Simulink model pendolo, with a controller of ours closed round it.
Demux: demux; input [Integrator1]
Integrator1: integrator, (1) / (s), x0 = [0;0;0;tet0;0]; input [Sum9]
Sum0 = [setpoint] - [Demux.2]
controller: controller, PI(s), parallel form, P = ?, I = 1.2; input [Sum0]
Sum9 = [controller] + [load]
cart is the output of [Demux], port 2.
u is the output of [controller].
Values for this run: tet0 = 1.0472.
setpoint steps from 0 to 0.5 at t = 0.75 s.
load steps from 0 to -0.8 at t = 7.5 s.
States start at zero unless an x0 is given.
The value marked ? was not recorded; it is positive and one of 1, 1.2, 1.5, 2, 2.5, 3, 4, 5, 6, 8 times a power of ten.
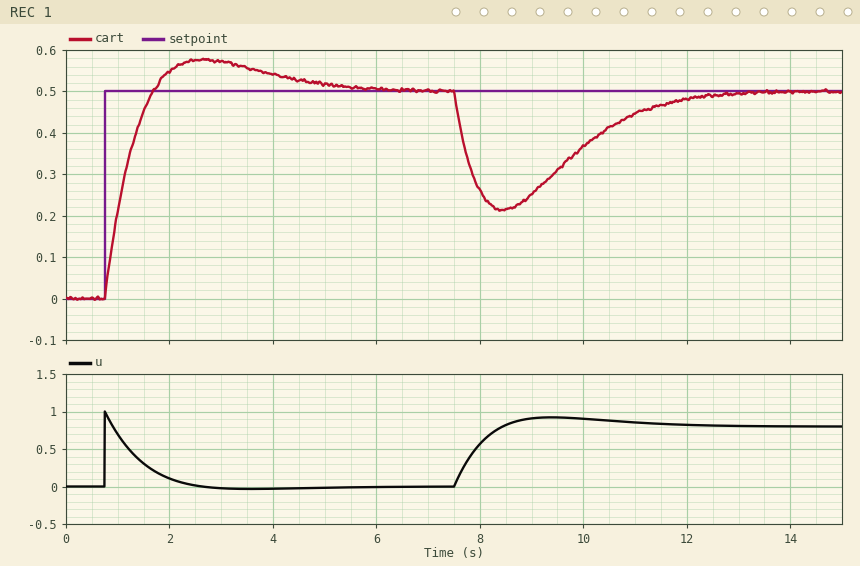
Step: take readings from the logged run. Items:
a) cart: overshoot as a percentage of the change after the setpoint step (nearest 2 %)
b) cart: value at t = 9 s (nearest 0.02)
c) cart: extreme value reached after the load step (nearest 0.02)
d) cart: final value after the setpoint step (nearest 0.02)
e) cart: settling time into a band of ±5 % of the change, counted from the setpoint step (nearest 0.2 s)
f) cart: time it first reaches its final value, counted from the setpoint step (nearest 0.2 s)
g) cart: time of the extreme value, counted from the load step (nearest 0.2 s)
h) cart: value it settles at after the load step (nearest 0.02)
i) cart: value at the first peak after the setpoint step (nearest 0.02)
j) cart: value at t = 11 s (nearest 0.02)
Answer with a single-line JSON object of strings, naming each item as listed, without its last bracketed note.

{"cart: overshoot as a percentage of the change after the setpoint step": "16 %", "cart: value at t = 9 s": "0.26", "cart: extreme value reached after the load step": "0.22", "cart: final value after the setpoint step": "0.50", "cart: settling time into a band of ±5 % of the change, counted from the setpoint step": "3.8 s", "cart: time it first reaches its final value, counted from the setpoint step": "1.0 s", "cart: time of the extreme value, counted from the load step": "1.0 s", "cart: value it settles at after the load step": "0.50", "cart: value at the first peak after the setpoint step": "0.58", "cart: value at t = 11 s": "0.44"}
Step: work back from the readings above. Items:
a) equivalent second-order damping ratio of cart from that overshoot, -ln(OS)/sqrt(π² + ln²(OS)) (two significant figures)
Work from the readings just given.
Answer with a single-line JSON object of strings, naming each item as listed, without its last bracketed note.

{"equivalent second-order damping ratio of cart from that overshoot, -ln(OS)/sqrt(π² + ln²(OS))": "0.50"}
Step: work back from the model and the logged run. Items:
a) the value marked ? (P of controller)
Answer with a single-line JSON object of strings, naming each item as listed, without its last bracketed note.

{"the value marked ?": "2"}
